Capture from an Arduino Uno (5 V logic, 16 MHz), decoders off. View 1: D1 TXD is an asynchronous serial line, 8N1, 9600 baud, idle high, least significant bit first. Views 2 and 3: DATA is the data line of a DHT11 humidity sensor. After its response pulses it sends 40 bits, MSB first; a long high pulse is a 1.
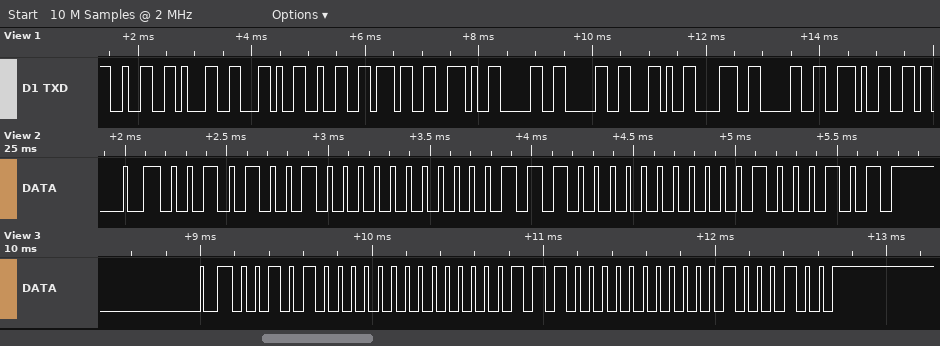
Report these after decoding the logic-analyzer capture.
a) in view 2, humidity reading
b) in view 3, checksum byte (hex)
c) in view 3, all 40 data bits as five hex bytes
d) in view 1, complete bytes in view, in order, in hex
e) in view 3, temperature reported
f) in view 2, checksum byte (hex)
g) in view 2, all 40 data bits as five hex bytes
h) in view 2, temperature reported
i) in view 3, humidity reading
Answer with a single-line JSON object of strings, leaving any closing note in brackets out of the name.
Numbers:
{"in view 2, humidity reading": "41 %", "in view 3, checksum byte": "0x44", "in view 3, all 40 data bits as five hex bytes": "28 00 1C 00 44", "in view 1, complete bytes in view, in order, in hex": "32 31 2C 32 37 2E 30 30 2C 38 30 2E", "in view 3, temperature reported": "28.0 °C", "in view 2, checksum byte": "0x45", "in view 2, all 40 data bits as five hex bytes": "29 00 1C 00 45", "in view 2, temperature reported": "28.0 °C", "in view 3, humidity reading": "40 %"}
